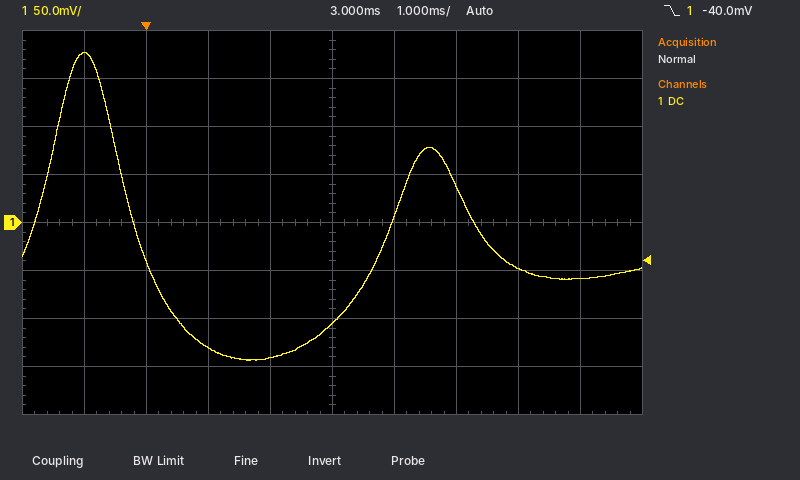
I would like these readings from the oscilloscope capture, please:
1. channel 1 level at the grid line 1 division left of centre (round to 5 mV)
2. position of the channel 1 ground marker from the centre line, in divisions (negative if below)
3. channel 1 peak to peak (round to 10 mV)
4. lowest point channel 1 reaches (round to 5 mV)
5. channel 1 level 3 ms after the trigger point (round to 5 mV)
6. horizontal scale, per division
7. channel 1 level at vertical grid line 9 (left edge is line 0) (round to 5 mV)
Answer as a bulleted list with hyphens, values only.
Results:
- -140 mV
- 0.0 div
- 320 mV
- -145 mV
- -105 mV
- 1 ms
- -60 mV
